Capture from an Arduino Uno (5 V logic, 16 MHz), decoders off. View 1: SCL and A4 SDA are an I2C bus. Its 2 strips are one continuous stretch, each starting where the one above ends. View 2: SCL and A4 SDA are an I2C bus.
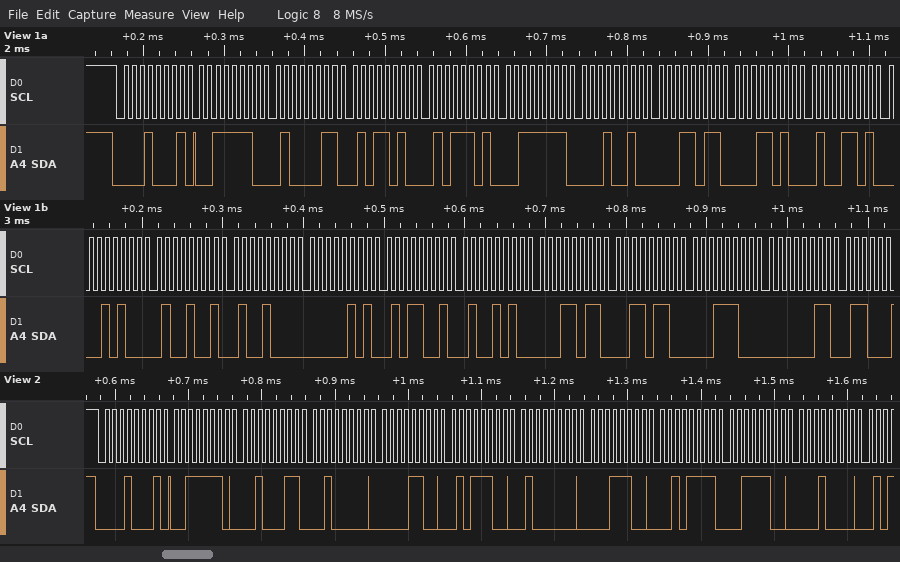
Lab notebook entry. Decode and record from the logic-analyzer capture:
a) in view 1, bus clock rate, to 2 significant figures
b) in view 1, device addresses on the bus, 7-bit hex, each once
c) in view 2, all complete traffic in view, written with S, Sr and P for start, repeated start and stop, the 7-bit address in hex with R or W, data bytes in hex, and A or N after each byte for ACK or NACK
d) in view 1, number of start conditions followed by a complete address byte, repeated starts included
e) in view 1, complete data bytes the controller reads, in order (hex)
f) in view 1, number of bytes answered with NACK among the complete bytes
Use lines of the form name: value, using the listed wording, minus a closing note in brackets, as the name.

in view 1, bus clock rate, to 2 significant figures: 100 kHz
in view 1, device addresses on the bus, 7-bit hex, each once: 0x08
in view 2, all complete traffic in view, written with S, Sr and P for start, repeated start and stop, the 7-bit address in hex with R or W, data bytes in hex, and A or N after each byte for ACK or NACK: S 08R A 3E A 23 A 20 A 0C A 5C A 40 A 1C A 2F A 3C A 10 A
in view 1, number of start conditions followed by a complete address byte, repeated starts included: 1
in view 1, complete data bytes the controller reads, in order: 3E 43 5A 5D 3F 12 1B 1A 4D 14 49 48 05 59 4A 1B 36 1C 03
in view 1, number of bytes answered with NACK among the complete bytes: 0
